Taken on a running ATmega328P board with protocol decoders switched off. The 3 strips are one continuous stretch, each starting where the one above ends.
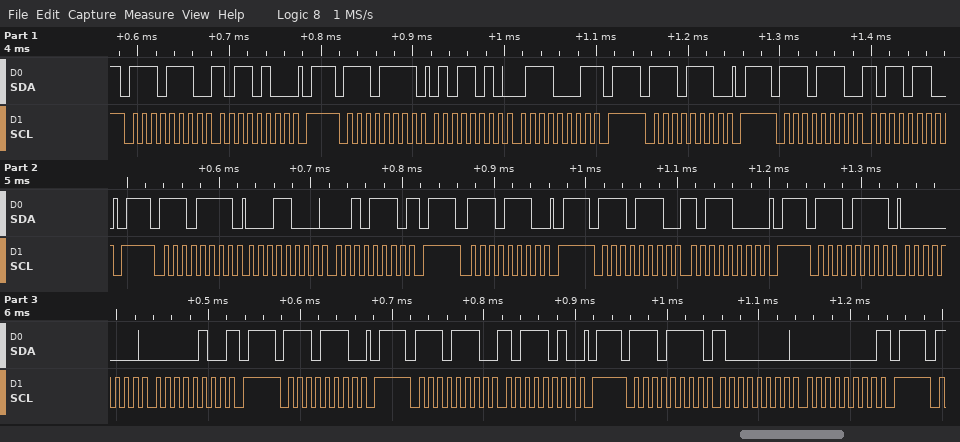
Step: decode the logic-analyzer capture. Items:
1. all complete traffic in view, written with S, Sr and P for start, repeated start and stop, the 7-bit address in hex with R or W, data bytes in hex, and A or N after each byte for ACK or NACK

S 77W A B4 A P S 77R A 5A A 71 N P S 77W A P S 77W A B6 A P S 77R A 18 A 2E N P S 77W A P S 77W A B8 A P S 77R A 00 A 04 N P S 77W A P S 77W A BA A P S 77R A 80 A 00 N P
